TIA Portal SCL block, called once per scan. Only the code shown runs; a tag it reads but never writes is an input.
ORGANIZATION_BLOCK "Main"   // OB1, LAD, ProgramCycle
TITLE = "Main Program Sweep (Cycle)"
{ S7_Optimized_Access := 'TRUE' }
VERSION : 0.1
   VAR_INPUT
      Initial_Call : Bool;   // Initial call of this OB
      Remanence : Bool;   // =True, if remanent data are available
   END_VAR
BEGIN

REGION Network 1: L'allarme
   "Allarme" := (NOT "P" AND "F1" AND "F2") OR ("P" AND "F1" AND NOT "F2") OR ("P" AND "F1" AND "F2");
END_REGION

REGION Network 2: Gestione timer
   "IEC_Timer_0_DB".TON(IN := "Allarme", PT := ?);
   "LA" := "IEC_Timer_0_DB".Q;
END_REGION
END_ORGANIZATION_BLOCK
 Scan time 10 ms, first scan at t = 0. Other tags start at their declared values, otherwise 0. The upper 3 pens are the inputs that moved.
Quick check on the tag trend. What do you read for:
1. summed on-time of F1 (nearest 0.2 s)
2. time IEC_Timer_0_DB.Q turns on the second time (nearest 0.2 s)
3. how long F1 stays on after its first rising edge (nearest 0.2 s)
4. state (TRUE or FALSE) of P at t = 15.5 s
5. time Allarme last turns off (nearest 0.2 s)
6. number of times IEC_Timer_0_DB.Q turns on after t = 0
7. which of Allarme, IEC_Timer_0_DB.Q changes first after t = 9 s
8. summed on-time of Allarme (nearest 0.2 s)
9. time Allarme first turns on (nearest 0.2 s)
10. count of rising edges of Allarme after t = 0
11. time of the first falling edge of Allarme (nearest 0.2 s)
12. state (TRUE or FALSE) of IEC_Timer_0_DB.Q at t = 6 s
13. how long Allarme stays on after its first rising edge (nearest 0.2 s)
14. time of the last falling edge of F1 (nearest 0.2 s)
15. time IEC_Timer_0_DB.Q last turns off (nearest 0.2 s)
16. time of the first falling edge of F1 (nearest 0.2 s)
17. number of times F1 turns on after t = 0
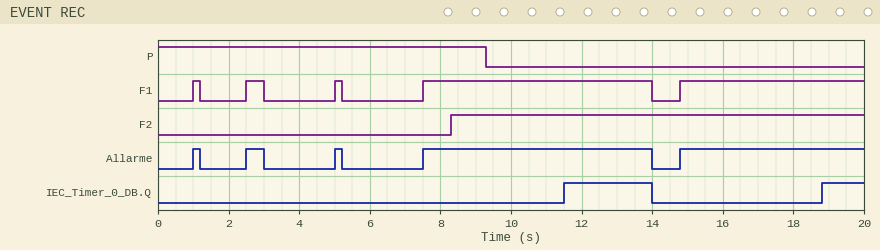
12.6 s
18.8 s
0.2 s
FALSE
14.0 s
2
IEC_Timer_0_DB.Q
12.6 s
1.0 s
5
1.2 s
FALSE
0.2 s
14.0 s
14.0 s
1.2 s
5
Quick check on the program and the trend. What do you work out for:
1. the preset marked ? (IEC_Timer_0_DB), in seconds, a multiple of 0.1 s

4.0 s
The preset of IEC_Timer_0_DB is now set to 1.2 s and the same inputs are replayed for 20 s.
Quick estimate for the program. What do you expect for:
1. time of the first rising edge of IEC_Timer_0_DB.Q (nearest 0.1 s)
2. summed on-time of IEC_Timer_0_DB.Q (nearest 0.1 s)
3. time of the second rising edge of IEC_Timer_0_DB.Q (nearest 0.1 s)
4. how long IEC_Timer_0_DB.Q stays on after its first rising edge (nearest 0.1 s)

8.7 s
9.3 s
16.0 s
5.3 s
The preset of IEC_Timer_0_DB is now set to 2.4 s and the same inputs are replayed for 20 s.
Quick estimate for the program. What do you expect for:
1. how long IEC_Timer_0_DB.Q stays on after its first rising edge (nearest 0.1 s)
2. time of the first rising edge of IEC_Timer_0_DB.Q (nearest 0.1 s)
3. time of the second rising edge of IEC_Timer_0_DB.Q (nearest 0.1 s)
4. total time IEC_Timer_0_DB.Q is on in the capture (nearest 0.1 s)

4.1 s
9.9 s
17.2 s
6.9 s
